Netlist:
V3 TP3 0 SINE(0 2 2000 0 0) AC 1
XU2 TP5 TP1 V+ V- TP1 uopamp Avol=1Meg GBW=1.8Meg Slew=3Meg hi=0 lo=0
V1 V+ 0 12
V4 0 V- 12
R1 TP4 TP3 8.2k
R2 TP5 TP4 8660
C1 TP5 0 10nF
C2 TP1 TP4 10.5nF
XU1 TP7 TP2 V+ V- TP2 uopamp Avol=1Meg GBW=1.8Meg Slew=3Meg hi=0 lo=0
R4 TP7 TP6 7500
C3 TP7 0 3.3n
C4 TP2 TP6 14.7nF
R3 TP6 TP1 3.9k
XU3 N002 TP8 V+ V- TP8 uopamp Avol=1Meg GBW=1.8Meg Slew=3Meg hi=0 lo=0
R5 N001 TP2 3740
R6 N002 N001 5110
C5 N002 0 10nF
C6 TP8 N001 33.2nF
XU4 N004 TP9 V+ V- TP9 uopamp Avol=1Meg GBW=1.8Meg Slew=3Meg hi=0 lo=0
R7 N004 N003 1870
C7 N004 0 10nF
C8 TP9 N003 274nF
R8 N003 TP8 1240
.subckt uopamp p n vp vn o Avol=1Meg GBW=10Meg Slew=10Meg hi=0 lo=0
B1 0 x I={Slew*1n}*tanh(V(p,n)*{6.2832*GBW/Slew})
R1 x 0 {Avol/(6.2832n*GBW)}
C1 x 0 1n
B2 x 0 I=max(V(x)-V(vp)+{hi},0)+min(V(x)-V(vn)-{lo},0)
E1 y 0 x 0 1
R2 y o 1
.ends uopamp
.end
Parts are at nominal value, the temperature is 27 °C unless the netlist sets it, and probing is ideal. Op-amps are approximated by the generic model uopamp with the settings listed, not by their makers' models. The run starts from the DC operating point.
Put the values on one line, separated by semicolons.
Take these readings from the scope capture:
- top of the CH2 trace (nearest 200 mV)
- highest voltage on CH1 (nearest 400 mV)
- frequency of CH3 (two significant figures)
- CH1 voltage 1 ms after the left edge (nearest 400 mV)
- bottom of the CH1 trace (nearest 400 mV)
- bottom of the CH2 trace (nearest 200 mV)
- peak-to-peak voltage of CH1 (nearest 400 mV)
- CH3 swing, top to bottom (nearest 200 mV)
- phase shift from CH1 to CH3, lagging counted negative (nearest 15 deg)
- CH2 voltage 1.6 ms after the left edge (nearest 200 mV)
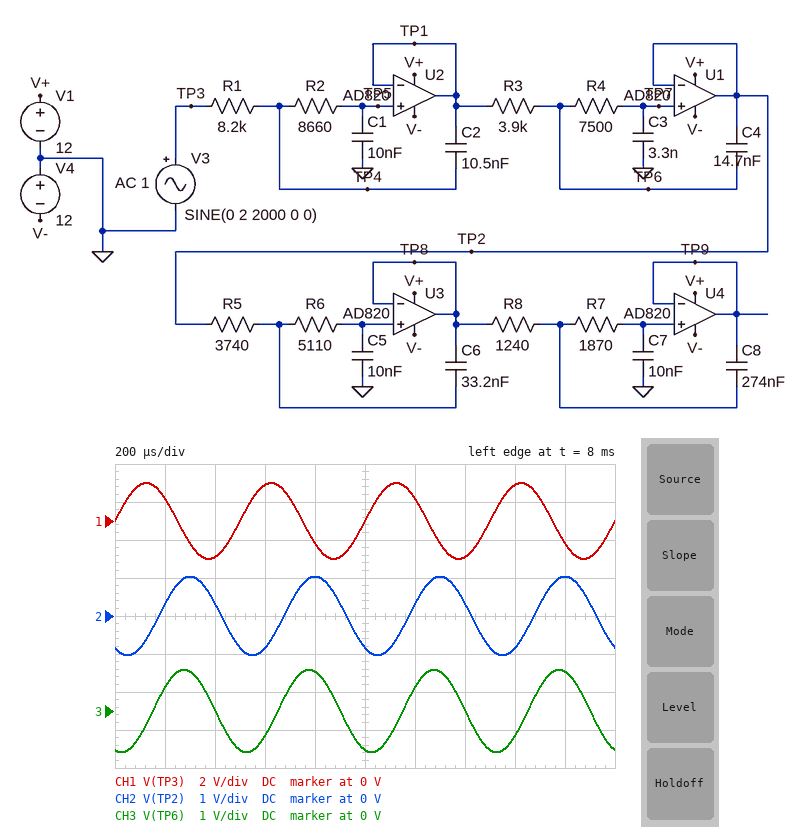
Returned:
1.0 V; 2.0 V; 2.0 kHz; 0 V; -2.0 V; -1.0 V; 4.0 V; 2.2 V; -105 deg; -800 mV
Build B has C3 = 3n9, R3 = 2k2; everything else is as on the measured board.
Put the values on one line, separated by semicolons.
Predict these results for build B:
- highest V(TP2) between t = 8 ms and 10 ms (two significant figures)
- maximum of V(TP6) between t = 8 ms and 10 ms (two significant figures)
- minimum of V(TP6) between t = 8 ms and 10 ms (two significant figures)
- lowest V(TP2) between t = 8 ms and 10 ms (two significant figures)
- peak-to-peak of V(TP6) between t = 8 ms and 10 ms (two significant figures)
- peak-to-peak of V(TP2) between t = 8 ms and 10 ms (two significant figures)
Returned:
970 mV; 1.0 V; -1.0 V; -970 mV; 2.1 V; 1.9 V
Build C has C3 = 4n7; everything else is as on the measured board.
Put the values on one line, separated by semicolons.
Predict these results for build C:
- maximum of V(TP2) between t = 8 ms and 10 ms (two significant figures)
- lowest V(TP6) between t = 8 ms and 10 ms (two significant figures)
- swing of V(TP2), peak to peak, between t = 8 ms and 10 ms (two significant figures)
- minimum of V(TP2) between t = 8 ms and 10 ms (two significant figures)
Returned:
980 mV; -1.1 V; 2.0 V; -980 mV
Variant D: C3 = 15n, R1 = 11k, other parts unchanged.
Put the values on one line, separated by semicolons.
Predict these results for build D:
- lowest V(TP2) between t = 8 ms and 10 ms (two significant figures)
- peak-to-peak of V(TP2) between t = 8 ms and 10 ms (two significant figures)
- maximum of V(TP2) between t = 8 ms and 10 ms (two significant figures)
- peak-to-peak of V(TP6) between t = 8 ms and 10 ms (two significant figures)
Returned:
-370 mV; 730 mV; 370 mV; 1.3 V
